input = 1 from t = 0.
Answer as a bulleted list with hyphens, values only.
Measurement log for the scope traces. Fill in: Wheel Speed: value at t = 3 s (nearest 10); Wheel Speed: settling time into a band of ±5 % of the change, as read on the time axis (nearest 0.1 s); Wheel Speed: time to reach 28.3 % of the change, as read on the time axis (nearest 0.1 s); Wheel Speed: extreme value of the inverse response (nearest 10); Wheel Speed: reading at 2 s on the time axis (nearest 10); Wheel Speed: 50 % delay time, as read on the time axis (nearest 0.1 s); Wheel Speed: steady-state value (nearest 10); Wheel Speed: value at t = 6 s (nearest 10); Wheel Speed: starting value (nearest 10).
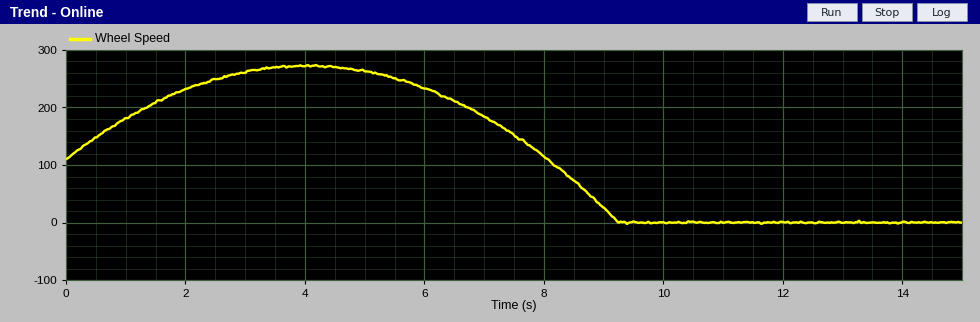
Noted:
- 260
- 9.2 s
- 8.4 s
- 270
- 230
- 8.7 s
- 0
- 230
- 110
